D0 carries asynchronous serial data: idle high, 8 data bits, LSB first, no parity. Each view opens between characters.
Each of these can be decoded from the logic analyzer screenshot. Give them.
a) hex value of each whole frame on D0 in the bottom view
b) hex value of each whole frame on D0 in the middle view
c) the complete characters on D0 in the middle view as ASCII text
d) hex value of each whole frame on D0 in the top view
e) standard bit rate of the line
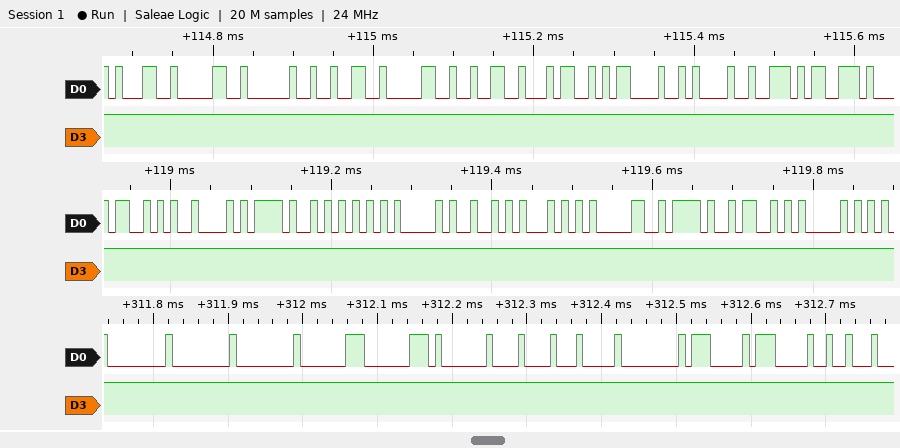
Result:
00, 00, 00, C0, C0, 01, 08, 04, 00, 07, 07, 12
53, 42, 2F, 55, 41, 52, 54, 30, 2F, 53, 50
"SB/UART0/SP"
31, 30, 20, 32, 30, 32, 34, 0D, 0A, 72, 73
115200 baud
